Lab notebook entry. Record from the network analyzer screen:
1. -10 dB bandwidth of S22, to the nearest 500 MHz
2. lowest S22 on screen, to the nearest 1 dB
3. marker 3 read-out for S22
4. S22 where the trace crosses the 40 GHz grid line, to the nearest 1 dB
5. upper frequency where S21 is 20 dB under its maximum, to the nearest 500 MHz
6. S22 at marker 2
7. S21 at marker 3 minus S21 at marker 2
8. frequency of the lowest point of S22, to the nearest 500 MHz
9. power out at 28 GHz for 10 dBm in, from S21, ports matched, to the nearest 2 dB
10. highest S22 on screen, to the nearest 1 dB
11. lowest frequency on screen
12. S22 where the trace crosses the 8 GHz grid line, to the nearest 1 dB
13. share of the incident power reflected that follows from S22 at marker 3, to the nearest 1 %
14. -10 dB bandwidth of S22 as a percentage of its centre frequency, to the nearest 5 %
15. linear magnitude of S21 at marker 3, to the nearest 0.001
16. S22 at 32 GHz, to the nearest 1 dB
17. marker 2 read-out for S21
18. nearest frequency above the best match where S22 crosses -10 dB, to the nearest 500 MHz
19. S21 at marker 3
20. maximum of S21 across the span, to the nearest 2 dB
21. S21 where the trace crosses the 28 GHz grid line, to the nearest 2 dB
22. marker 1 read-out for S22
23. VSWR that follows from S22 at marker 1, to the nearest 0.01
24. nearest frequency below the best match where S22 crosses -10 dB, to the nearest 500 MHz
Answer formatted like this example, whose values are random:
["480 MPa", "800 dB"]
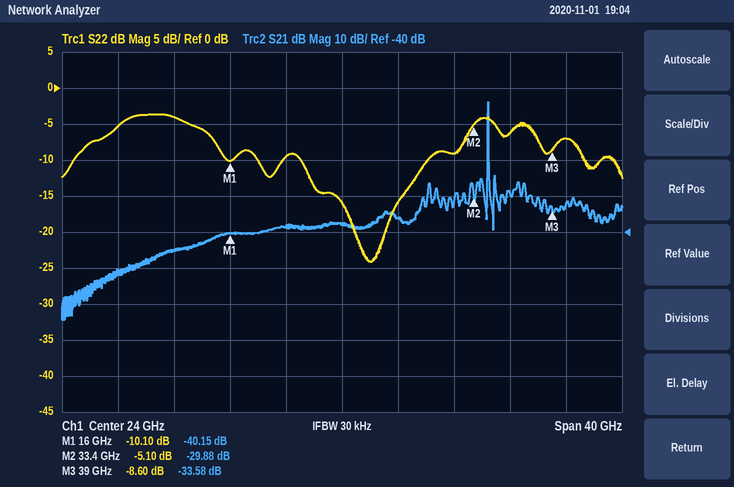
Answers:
["9.0 GHz", "-24 dB", "-8.60 dB", "-7 dB", "34.5 GHz", "-5.10 dB", "-3.70 dB", "26.0 GHz", "-26 dBm", "-4 dB", "4 GHz", "-5 dB", "14 %", "35 %", "0.021", "-9 dB", "-29.88 dB", "30.0 GHz", "-33.58 dB", "-4 dB", "-36 dB", "-10.10 dB", "1.91", "21.0 GHz"]
